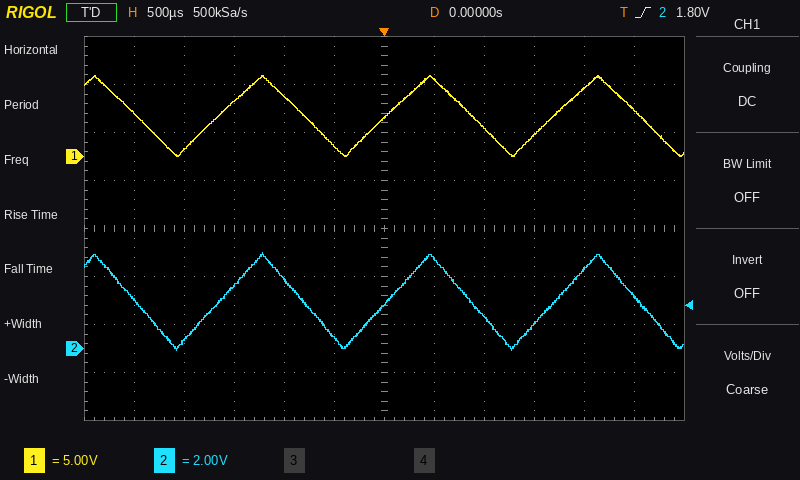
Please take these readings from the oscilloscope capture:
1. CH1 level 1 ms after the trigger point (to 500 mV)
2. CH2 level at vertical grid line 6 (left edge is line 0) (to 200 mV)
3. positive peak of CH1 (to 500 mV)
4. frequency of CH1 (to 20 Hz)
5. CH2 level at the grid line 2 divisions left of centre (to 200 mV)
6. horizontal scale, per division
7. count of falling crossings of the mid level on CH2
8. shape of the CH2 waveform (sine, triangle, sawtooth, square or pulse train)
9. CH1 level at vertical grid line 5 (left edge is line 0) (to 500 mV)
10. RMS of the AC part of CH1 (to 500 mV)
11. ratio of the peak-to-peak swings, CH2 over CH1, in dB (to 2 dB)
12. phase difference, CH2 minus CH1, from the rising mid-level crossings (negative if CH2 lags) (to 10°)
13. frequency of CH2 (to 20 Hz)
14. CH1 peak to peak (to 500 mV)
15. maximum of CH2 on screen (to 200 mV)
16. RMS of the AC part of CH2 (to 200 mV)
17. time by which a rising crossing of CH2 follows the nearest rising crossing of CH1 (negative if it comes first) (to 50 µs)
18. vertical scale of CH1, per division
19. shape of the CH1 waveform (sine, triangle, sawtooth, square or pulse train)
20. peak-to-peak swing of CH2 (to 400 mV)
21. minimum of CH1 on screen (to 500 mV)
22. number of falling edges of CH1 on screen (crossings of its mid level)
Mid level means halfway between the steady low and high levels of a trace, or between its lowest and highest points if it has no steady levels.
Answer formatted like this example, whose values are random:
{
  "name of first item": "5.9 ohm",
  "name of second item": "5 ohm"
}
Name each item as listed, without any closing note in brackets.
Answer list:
{
  "CH1 level 1 ms after the trigger point": "3.0 V",
  "CH2 level at vertical grid line 6 (left edge is line 0)": "1.8 V",
  "positive peak of CH1": "8.5 V",
  "frequency of CH1": "600 Hz",
  "CH2 level at the grid line 2 divisions left of centre": "2.8 V",
  "horizontal scale, per division": "500 µs",
  "count of falling crossings of the mid level on CH2": "4",
  "shape of the CH2 waveform": "triangle",
  "CH1 level at vertical grid line 5 (left edge is line 0)": "1.0 V",
  "RMS of the AC part of CH1": "2.5 V",
  "ratio of the peak-to-peak swings, CH2 over CH1, in dB": "-6 dB",
  "phase difference, CH2 minus CH1, from the rising mid-level crossings (negative if CH2 lags)": "0°",
  "frequency of CH2": "600 Hz",
  "CH1 peak to peak": "8.5 V",
  "maximum of CH2 on screen": "4.0 V",
  "RMS of the AC part of CH2": "1.2 V",
  "time by which a rising crossing of CH2 follows the nearest rising crossing of CH1 (negative if it comes first)": "0 µs",
  "vertical scale of CH1, per division": "5 V",
  "shape of the CH1 waveform": "triangle",
  "peak-to-peak swing of CH2": "4.0 V",
  "minimum of CH1 on screen": "0.0 V",
  "number of falling edges of CH1 on screen": "4"
}
